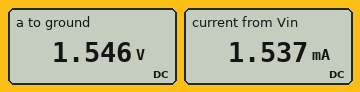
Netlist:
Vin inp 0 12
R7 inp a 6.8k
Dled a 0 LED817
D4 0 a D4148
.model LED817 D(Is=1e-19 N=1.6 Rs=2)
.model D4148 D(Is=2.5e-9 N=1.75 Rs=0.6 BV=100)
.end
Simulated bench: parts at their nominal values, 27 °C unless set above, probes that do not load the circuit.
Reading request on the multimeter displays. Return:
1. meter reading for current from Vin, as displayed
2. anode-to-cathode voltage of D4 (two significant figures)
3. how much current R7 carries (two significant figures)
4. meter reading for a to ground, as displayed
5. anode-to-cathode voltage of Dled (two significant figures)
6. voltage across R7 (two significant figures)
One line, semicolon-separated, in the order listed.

1.537 mA; -1.5 V; 1.5 mA; 1.546 V; 1.5 V; 10 V
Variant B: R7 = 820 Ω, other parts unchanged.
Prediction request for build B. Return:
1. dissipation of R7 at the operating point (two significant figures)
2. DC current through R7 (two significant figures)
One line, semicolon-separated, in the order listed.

130 mW; 13 mA
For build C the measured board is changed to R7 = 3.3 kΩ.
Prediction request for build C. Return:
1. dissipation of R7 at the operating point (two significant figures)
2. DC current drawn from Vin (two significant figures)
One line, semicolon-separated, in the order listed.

33 mW; 3.2 mA
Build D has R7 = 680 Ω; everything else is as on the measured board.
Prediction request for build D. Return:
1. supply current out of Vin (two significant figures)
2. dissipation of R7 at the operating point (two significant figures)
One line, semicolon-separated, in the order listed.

15 mA; 160 mW
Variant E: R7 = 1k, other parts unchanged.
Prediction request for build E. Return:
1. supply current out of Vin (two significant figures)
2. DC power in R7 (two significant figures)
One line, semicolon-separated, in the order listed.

10 mA; 110 mW
